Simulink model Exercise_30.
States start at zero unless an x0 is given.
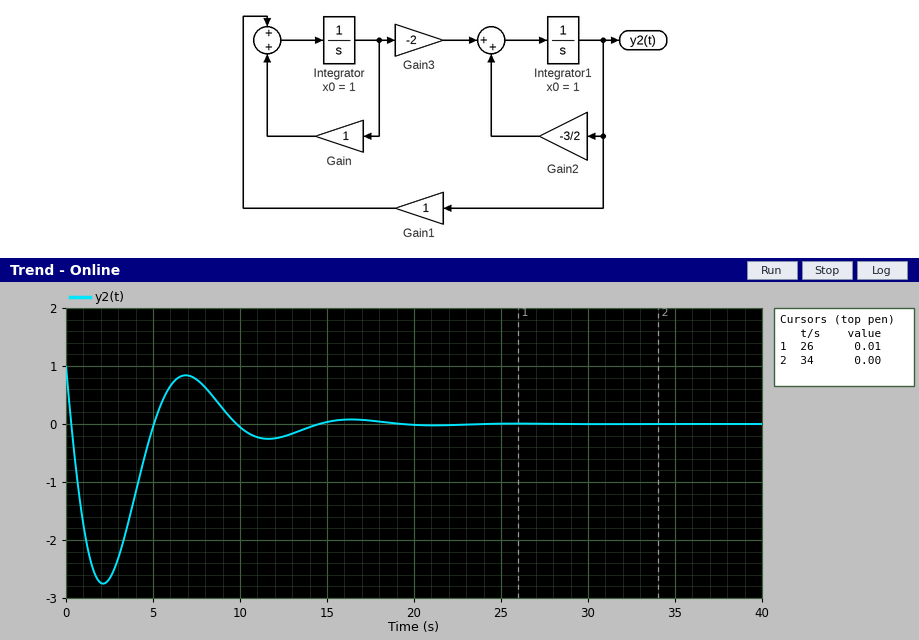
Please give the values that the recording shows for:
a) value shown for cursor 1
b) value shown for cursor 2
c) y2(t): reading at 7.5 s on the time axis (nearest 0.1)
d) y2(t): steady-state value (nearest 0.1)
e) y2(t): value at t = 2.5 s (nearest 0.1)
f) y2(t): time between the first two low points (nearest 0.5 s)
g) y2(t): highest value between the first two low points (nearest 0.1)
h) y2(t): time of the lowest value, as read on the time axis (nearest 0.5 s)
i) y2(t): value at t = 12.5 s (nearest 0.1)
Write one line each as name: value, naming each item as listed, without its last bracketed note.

value shown for cursor 1: 0.01
value shown for cursor 2: 0.00
y2(t): reading at 7.5 s on the time axis: 0.8
y2(t): steady-state value: 0.0
y2(t): value at t = 2.5 s: -2.7
y2(t): time between the first two low points: 9.5 s
y2(t): highest value between the first two low points: 0.8
y2(t): time of the lowest value, as read on the time axis: 2.0 s
y2(t): value at t = 12.5 s: -0.2
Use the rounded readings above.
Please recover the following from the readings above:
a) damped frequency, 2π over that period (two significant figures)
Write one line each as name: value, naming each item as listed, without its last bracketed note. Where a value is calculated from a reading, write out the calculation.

damped frequency, 2π over that period: 2π / 9.5 = 0.66 rad/s
